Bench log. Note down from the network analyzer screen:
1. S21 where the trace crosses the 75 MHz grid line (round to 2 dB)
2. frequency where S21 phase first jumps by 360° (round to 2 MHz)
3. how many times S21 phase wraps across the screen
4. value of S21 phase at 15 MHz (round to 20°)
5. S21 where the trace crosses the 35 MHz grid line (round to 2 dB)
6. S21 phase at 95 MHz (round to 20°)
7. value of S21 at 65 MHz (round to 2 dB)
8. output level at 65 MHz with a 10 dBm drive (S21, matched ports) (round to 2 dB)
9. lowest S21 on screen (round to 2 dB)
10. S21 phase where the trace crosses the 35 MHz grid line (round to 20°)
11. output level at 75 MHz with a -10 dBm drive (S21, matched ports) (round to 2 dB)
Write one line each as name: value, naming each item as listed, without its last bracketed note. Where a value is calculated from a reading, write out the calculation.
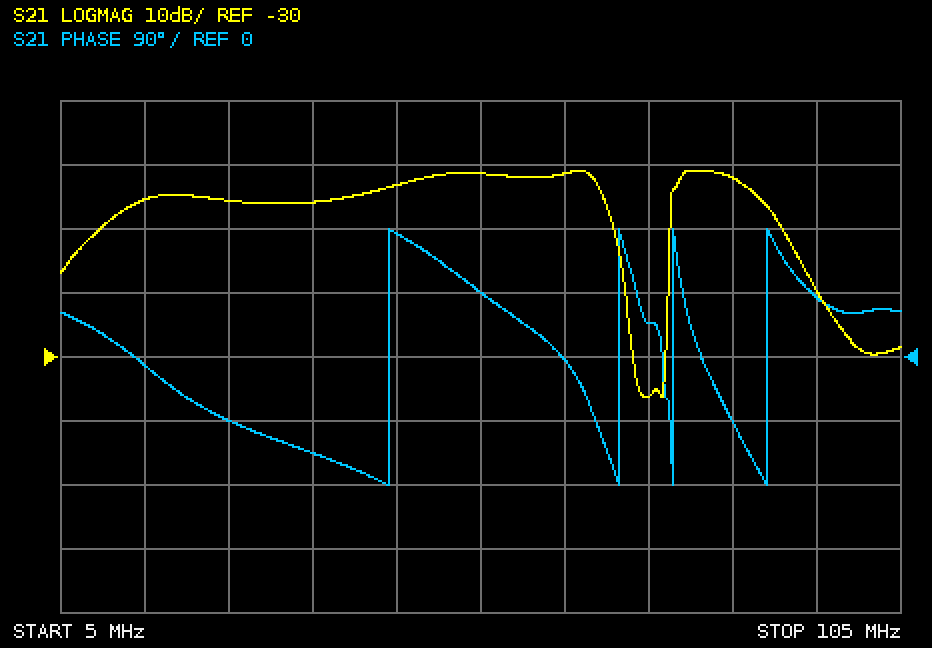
S21 where the trace crosses the 75 MHz grid line: -36 dB
frequency where S21 phase first jumps by 360°: 44 MHz
how many times S21 phase wraps across the screen: 4
value of S21 phase at 15 MHz: -20°
S21 where the trace crosses the 35 MHz grid line: -6 dB
S21 phase at 95 MHz: 80°
value of S21 at 65 MHz: -2 dB
output level at 65 MHz with a 10 dBm drive (S21, matched ports): 10 dBm + (-2 dB) = 8 dBm
lowest S21 on screen: -36 dB
S21 phase where the trace crosses the 35 MHz grid line: -140°
output level at 75 MHz with a -10 dBm drive (S21, matched ports): -10 dBm + (-36 dB) = -46 dBm
